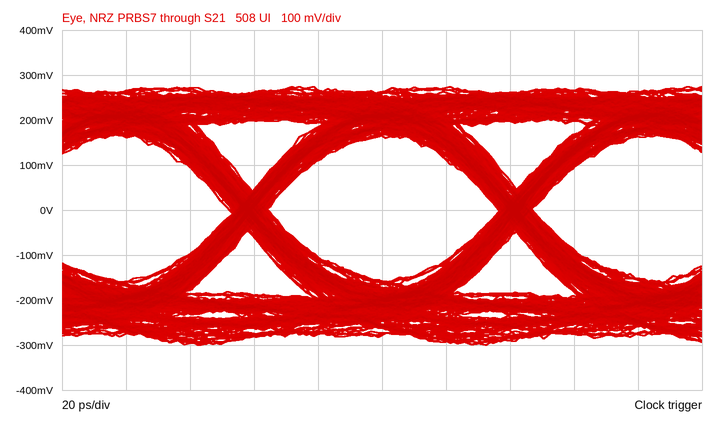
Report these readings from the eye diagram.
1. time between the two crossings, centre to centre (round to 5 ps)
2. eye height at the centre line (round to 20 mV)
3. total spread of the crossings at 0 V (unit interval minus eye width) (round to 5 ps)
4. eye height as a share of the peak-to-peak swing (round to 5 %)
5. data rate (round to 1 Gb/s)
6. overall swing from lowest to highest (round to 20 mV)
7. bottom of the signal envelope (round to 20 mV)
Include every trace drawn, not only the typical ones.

85 ps
320 mV
10 ps
55 %
12 Gb/s
580 mV
-300 mV
